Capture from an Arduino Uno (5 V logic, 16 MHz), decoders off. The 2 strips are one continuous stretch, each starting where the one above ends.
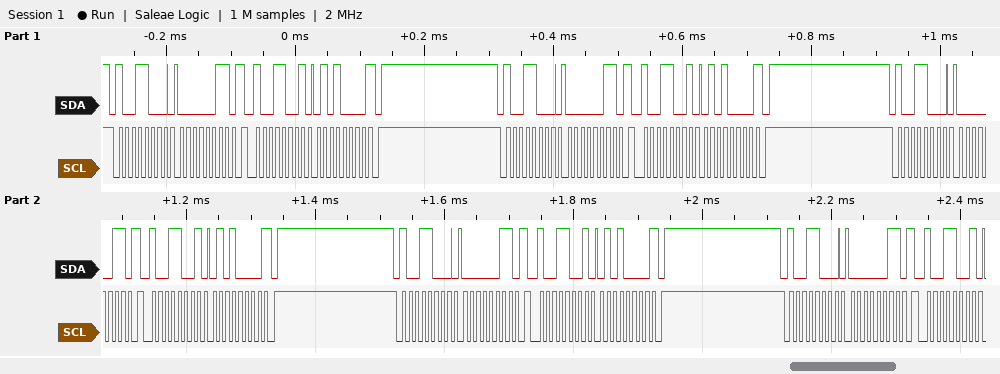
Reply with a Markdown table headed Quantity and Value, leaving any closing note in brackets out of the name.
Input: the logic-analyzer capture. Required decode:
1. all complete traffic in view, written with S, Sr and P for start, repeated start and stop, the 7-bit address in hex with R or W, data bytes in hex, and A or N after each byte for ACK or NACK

| Quantity | Value |
|---|---|
| all complete traffic in view, written with S, Sr and P for start, repeated start and stop, the 7-bit address in hex with R or W, data bytes in hex, and A or N after each byte for ACK or NACK | S 4CW A 03 A Sr 4CR A 50 N P S 4CW A 03 A Sr 4CR A 50 N P S 4CW A 03 A Sr 4CR A 50 N P S 4CW A 03 A Sr 4CR A 50 N P S 4CW A 03 A Sr 4CR A |
